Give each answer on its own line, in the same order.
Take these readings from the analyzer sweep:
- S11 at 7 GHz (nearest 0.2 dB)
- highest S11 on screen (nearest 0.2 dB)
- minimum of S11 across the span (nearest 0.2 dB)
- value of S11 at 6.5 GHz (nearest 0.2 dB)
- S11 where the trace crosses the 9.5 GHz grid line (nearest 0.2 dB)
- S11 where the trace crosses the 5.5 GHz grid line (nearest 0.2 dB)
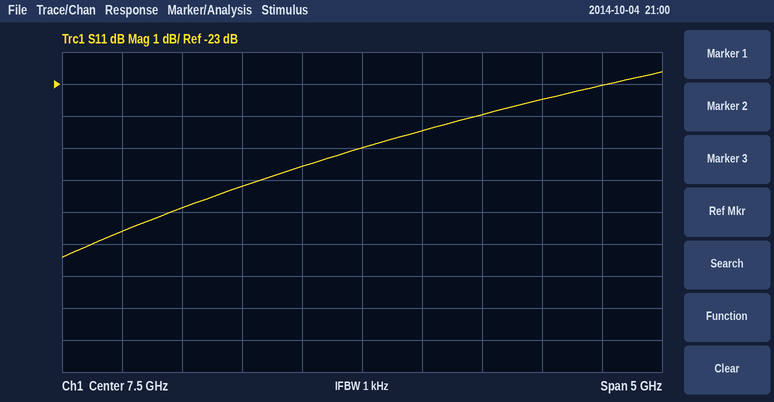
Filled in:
-25.6 dB
-22.6 dB
-28.4 dB
-26.2 dB
-23.0 dB
-27.6 dB
